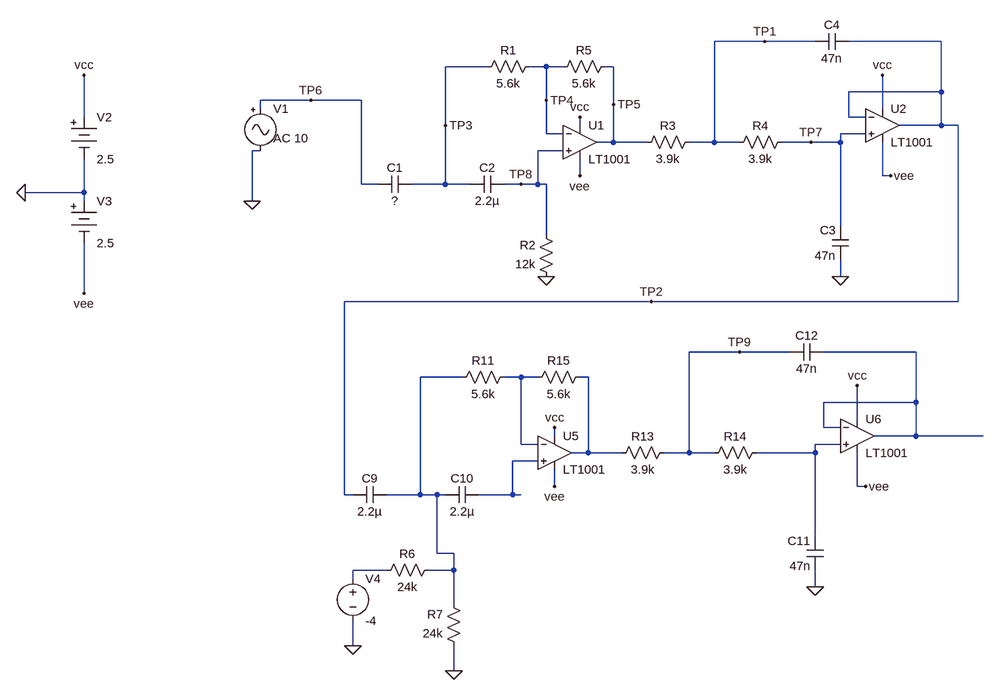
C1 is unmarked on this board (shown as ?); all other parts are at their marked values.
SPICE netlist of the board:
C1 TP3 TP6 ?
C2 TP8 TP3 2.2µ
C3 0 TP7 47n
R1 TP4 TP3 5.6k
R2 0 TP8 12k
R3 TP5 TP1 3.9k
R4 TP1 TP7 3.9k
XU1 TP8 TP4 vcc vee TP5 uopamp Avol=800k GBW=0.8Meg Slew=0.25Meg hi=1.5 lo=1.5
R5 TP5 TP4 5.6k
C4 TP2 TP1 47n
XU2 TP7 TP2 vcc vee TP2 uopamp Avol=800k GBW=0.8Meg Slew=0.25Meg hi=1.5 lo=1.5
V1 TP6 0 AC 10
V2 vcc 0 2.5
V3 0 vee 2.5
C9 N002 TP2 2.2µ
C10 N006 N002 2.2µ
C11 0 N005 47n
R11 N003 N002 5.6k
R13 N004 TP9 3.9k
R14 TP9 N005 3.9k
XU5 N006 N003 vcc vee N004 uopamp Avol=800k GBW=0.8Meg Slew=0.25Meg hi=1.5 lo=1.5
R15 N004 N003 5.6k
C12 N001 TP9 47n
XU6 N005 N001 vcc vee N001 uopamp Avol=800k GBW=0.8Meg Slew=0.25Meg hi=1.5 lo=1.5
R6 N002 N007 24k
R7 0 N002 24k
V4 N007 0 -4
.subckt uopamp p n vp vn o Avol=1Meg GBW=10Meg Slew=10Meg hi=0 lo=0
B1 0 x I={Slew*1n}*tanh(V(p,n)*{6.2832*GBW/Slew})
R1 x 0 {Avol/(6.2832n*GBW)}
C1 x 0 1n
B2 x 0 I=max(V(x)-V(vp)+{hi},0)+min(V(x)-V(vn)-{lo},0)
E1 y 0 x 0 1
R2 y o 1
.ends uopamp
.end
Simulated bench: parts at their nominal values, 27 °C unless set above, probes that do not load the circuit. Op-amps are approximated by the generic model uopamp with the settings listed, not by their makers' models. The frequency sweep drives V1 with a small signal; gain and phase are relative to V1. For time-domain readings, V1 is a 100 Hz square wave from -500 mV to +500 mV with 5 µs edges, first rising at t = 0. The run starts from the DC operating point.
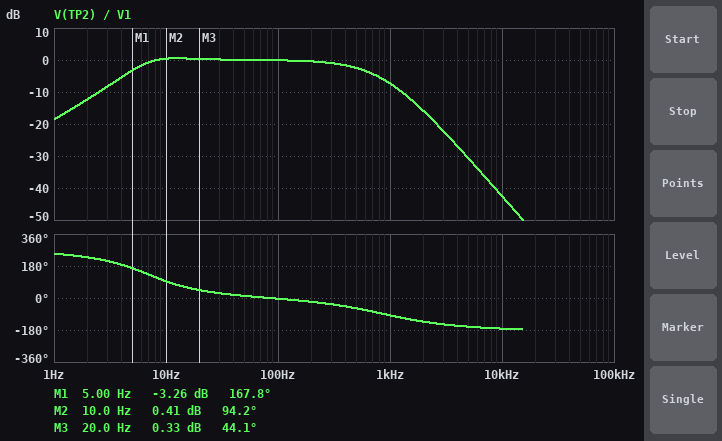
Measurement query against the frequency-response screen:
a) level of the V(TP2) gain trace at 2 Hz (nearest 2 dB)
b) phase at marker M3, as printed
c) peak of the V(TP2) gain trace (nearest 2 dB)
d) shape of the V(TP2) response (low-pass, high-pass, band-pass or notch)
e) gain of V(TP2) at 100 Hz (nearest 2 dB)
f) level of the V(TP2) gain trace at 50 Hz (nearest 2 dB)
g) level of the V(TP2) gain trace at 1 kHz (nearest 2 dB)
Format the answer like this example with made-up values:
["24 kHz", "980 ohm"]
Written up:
["-12 dB", "44.1 deg", "0 dB", "band-pass", "0 dB", "0 dB", "-8 dB"]
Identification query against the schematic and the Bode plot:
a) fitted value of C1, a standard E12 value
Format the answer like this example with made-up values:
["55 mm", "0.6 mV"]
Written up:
["3.3 µF"]
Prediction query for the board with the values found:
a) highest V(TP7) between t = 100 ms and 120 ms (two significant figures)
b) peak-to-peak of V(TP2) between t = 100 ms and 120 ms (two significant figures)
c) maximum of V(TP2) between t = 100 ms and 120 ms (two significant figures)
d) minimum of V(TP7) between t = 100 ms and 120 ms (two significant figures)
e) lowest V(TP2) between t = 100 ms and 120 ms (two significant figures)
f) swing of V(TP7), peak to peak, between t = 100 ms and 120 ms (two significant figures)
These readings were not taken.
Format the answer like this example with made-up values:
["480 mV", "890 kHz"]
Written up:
["570 mV", "1.1 V", "570 mV", "-570 mV", "-570 mV", "1.1 V"]
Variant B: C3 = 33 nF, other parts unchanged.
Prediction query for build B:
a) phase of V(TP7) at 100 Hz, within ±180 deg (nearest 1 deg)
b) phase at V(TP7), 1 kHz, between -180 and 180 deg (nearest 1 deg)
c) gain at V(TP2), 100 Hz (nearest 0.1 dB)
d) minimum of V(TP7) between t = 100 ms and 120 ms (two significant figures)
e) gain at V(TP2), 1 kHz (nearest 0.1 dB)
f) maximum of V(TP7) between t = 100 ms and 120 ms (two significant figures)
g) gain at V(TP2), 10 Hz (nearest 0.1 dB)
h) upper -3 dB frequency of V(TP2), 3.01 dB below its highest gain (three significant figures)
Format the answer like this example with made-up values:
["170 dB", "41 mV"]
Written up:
["0 deg", "-87 deg", "0 dB", "-600 mV", "-4.2 dB", "610 mV", "0.4 dB", "778 Hz"]
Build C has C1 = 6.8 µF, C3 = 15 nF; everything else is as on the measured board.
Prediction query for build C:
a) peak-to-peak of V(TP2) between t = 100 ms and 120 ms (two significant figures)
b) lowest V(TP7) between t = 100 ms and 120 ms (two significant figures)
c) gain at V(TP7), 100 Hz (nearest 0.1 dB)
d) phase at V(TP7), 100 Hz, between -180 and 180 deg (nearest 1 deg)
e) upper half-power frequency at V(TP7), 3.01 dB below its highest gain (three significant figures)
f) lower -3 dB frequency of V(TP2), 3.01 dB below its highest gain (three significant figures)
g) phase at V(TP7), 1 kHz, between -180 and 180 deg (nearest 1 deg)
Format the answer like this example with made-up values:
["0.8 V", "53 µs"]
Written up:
["1.4 V", "-710 mV", "0 dB", "4 deg", "1.75 kHz", "3.31 Hz", "-51 deg"]
